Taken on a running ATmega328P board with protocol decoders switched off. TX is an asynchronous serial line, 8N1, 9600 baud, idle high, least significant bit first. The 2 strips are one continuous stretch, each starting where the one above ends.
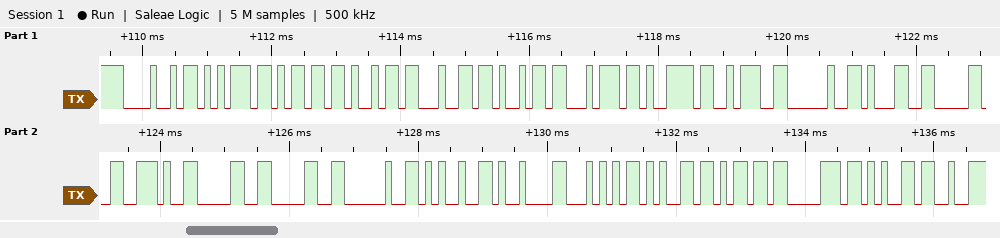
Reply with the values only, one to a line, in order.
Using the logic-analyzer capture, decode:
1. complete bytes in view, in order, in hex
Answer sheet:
48 75 6D 69 64 69 74 79 3A 20 31 30 2E 30 30 20 25 09 54 65 6D 70 65
